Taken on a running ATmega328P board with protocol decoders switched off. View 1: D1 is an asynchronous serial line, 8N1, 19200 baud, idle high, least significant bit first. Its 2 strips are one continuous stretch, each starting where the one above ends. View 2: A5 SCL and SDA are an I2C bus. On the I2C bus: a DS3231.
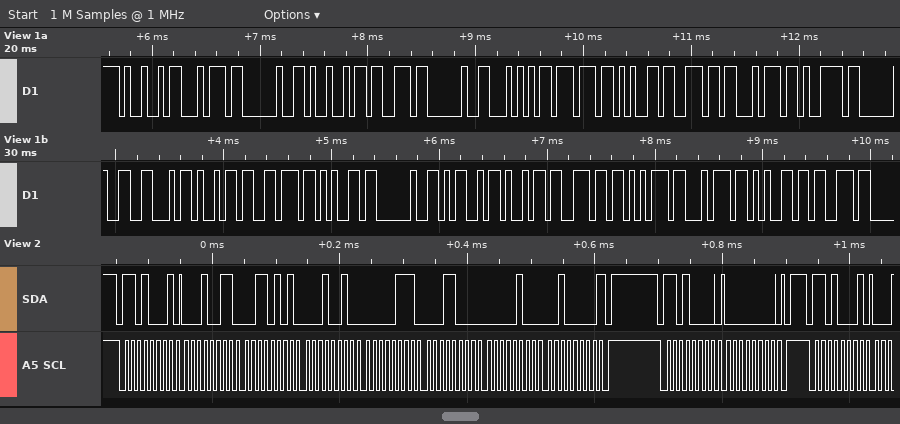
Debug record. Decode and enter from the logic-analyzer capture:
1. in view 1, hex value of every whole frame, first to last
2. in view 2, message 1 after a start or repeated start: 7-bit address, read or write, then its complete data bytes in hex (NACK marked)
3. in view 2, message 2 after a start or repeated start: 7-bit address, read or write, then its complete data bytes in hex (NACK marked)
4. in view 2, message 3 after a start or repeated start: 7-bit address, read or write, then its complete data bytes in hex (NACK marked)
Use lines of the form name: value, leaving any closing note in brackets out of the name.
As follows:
in view 1, hex value of every whole frame, first to last: 49 74 20 49 73 20 54 77 65 6E 74 79 20 46 69 76 65 20 4D 69 6E 75 74 65 73
in view 2, message 1 after a start or repeated start: 7-bit address, read or write, then its complete data bytes in hex: 0x68 read: 13 35 12 07 18 04 20 NACK
in view 2, message 2 after a start or repeated start: 7-bit address, read or write, then its complete data bytes in hex: 0x68 write: 00
in view 2, message 3 after a start or repeated start: 7-bit address, read or write, then its complete data bytes in hex: 0x68 read
